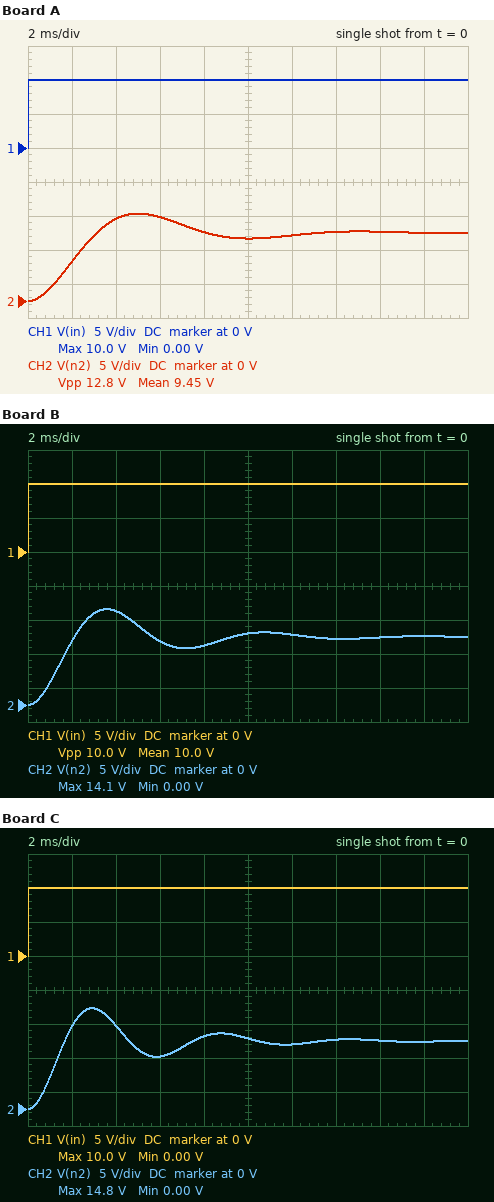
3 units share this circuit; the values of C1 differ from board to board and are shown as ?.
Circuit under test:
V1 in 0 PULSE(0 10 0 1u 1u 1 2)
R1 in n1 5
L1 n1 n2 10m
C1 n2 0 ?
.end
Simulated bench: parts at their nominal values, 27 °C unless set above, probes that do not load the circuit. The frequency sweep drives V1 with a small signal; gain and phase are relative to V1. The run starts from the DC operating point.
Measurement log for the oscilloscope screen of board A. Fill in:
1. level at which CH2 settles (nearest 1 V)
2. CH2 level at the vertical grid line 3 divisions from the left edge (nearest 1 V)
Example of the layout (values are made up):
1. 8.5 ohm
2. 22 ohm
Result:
1. 10 V
2. 12 V
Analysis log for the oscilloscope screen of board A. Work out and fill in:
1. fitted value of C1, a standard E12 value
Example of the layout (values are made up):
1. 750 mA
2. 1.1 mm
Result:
1. 220 µF
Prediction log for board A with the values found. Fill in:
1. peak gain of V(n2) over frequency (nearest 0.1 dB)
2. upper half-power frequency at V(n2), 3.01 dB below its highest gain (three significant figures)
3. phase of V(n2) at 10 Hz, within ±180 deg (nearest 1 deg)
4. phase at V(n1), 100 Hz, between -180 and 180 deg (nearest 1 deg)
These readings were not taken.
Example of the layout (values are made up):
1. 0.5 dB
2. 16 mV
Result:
1. 3.2 dB
2. 128 Hz
3. -4 deg
4. -79 deg
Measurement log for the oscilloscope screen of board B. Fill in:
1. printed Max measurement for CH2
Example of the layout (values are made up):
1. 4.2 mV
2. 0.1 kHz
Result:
1. 14.1 V
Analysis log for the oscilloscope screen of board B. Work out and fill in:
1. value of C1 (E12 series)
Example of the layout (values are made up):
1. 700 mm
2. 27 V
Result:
1. 120 µF
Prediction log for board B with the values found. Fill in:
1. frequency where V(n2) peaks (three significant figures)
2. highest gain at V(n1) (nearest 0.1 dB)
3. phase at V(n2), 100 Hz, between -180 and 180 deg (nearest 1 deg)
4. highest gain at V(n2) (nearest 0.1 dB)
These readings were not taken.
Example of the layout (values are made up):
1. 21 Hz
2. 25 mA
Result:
1. 134 Hz
2. 0 dB
3. -36 deg
4. 5.6 dB
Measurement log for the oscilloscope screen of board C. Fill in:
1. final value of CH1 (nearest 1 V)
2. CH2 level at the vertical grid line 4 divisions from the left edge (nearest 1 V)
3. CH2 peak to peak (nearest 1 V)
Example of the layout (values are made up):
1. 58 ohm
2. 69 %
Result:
1. 10 V
2. 11 V
3. 15 V
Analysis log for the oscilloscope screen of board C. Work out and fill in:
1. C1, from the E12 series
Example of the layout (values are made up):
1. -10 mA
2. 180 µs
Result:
1. 82 µF
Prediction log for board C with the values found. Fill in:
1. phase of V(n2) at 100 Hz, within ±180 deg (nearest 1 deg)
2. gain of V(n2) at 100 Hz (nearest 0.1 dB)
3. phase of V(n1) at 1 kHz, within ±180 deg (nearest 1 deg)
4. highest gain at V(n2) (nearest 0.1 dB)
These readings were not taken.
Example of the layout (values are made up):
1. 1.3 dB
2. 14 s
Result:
1. -21 deg
2. 2.8 dB
3. 5 deg
4. 7.1 dB
